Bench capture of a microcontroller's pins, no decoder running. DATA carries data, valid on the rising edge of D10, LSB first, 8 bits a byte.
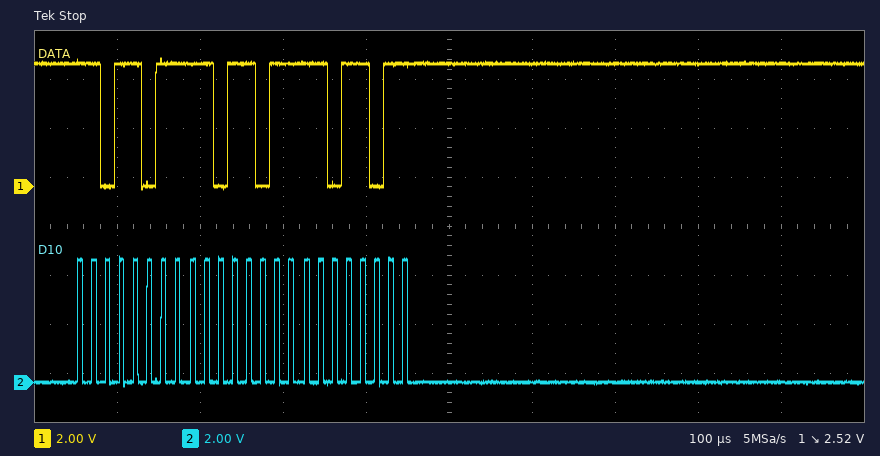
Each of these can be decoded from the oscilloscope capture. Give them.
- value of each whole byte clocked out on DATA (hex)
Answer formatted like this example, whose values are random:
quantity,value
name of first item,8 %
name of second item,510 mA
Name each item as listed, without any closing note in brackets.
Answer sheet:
quantity,value
value of each whole byte clocked out on DATA,0xDB 0xDB 0xDB
